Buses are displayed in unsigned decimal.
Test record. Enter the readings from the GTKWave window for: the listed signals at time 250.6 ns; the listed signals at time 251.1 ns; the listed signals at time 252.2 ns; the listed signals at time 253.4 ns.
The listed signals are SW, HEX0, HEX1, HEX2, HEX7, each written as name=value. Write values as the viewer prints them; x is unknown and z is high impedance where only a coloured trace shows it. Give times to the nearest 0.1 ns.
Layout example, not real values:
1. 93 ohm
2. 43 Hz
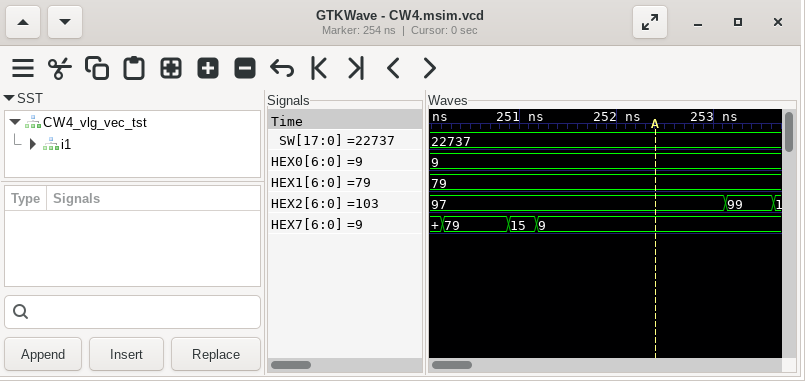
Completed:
1. SW=22737, HEX0=9, HEX1=79, HEX2=97, HEX7=79
2. SW=22737, HEX0=9, HEX1=79, HEX2=97, HEX7=15
3. SW=22737, HEX0=9, HEX1=79, HEX2=97, HEX7=9
4. SW=22737, HEX0=9, HEX1=79, HEX2=99, HEX7=9
